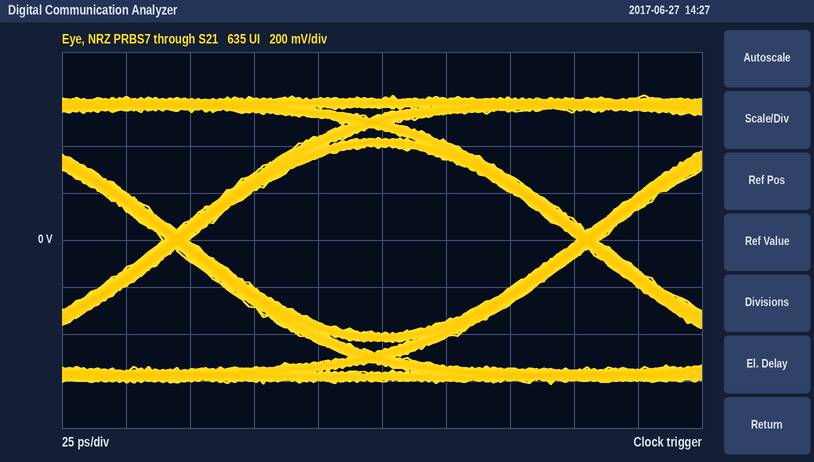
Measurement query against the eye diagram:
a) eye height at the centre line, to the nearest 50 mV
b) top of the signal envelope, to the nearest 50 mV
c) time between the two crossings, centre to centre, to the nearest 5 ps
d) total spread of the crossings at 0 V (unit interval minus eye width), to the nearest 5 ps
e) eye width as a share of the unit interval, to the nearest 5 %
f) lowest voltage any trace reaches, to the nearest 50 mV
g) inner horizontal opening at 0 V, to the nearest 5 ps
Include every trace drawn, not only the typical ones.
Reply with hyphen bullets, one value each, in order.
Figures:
- 800 mV
- 600 mV
- 160 ps
- 10 ps
- 95 %
- -600 mV
- 150 ps
